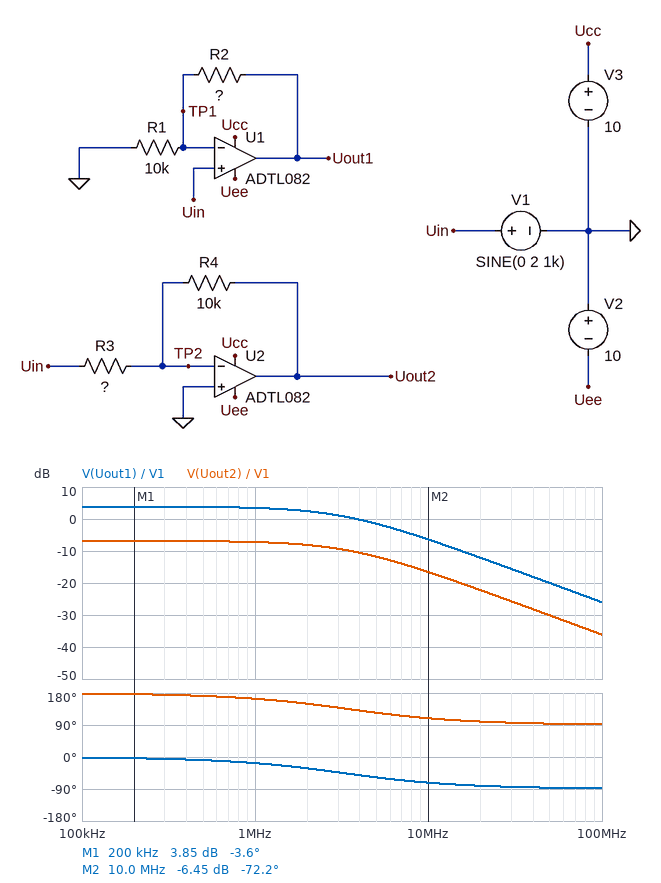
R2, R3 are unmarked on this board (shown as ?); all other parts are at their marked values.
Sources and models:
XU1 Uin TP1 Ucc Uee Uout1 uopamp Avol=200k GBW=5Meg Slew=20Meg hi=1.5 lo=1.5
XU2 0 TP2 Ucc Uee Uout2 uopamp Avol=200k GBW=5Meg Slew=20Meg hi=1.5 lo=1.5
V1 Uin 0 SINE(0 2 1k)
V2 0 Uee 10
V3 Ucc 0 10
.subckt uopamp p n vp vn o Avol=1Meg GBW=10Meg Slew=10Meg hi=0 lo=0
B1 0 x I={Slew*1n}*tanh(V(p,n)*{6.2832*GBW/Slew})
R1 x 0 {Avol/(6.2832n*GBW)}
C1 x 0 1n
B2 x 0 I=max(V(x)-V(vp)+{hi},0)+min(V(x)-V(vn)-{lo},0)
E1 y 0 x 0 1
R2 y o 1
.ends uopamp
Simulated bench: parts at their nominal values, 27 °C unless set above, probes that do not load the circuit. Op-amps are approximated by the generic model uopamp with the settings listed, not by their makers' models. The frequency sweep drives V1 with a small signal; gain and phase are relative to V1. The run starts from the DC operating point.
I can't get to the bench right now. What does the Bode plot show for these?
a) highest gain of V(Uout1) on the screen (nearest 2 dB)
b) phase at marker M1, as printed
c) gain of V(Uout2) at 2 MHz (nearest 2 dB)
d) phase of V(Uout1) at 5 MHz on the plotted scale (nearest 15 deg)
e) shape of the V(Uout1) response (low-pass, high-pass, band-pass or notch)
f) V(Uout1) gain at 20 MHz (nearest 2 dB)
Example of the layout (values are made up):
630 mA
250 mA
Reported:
4 dB
-3.6 deg
-8 dB
-60 deg
low-pass
-12 dB
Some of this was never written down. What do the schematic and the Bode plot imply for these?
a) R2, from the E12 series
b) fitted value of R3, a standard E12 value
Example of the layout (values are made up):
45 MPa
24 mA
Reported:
5.6 kΩ
22 kΩ
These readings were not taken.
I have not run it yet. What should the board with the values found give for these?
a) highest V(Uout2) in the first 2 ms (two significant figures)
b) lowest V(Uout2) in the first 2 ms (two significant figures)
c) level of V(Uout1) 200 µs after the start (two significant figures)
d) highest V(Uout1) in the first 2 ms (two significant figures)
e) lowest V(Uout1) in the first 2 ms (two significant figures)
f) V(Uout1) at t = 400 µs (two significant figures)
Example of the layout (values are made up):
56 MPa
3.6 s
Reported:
910 mV
-910 mV
3.0 V
3.1 V
-3.1 V
1.8 V
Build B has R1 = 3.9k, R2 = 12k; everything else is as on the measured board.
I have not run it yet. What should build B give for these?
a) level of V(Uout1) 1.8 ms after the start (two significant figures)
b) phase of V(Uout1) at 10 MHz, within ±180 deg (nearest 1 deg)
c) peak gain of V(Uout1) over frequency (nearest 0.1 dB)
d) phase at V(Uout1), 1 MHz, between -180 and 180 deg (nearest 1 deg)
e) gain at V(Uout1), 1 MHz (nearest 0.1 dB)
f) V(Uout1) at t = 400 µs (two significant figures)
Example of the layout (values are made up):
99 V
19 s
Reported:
-7.8 V
-83 deg
12.2 dB
-39 deg
10.0 dB
4.8 V
